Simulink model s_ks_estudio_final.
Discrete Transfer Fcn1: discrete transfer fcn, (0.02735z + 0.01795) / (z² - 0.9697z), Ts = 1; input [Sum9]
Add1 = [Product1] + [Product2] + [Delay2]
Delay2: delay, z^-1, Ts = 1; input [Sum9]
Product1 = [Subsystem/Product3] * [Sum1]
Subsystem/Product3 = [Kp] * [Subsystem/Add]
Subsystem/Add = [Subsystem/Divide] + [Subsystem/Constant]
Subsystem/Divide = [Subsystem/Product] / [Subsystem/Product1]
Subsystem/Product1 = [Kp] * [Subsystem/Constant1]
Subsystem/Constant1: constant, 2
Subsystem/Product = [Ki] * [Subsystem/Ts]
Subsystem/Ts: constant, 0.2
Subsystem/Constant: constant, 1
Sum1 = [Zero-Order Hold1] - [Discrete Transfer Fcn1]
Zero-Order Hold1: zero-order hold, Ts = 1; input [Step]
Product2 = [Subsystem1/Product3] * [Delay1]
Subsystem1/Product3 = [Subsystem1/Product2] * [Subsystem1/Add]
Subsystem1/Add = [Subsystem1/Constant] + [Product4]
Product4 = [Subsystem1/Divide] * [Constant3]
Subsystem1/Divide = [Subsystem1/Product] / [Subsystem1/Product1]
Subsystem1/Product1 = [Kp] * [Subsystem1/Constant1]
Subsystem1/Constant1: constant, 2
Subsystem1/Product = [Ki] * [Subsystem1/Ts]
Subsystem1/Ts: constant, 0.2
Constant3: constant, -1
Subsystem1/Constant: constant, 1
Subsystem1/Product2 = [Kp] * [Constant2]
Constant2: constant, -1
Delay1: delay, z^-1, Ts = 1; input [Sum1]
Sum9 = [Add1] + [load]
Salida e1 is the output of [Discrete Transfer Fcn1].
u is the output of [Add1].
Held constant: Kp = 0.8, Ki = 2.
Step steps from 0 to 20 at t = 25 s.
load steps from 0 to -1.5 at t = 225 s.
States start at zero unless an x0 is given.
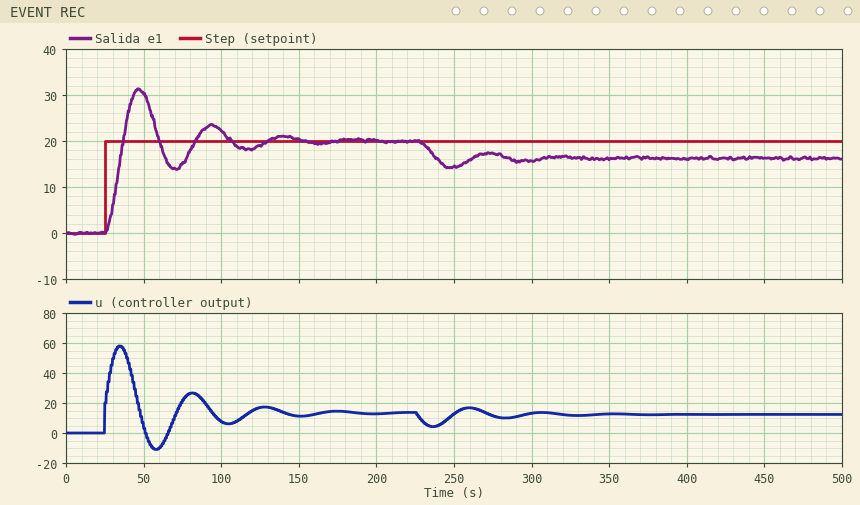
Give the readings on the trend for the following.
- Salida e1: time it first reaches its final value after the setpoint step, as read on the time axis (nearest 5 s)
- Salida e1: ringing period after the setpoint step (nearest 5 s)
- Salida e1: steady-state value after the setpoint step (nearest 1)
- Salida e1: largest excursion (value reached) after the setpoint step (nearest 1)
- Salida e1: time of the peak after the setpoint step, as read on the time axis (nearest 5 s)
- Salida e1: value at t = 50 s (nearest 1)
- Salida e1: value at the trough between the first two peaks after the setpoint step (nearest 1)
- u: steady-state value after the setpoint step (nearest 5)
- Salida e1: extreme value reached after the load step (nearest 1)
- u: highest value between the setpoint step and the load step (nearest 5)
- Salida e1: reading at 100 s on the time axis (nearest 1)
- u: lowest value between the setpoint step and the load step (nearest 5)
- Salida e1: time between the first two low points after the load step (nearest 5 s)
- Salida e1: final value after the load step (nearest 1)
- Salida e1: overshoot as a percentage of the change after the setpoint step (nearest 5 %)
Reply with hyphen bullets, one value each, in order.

- 35 s
- 45 s
- 20
- 31
- 45 s
- 30
- 14
- 15
- 14
- 60
- 22
- -10
- 45 s
- 16
- 55 %
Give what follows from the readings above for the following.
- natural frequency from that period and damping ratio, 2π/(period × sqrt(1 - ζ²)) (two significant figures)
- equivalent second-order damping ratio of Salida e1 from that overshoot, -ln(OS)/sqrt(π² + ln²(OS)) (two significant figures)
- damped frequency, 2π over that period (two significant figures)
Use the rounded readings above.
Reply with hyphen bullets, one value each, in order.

- 0.14 rad/s
- 0.19
- 0.14 rad/s
